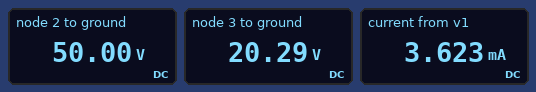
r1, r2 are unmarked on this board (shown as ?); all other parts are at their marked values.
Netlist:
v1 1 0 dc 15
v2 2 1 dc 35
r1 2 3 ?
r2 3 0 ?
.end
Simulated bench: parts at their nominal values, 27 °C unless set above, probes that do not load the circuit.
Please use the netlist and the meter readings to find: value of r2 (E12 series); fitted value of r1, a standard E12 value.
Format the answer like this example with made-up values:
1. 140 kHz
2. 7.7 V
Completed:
1. 5.6 kΩ
2. 8.2 kΩ
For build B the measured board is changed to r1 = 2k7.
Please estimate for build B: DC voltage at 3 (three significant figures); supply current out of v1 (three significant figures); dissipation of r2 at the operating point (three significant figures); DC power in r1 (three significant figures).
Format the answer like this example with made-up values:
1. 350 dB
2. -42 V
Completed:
1. 33.7 V
2. 6.02 mA
3. 203 mW
4. 98.0 mW
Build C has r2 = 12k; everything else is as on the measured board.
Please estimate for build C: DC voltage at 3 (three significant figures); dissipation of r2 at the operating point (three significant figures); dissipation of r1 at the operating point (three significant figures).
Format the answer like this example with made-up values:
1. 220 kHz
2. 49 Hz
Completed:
1. 29.7 V
2. 73.5 mW
3. 50.2 mW
